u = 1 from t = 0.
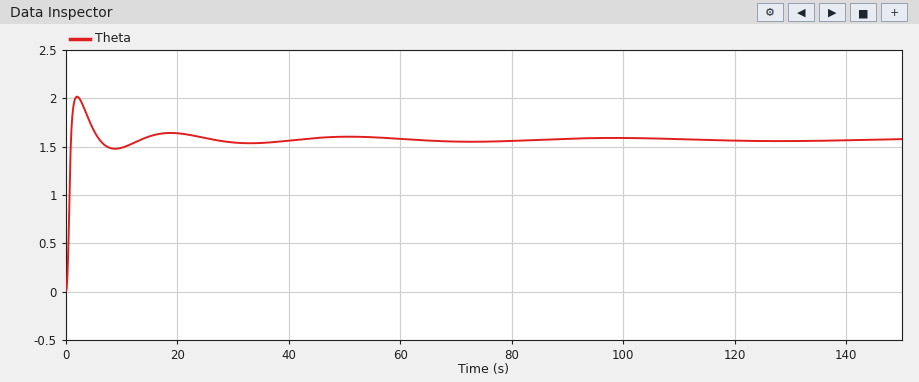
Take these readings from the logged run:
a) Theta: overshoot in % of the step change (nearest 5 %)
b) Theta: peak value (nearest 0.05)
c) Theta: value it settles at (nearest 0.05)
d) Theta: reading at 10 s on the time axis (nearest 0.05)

30 %
2.00
1.55
1.50
